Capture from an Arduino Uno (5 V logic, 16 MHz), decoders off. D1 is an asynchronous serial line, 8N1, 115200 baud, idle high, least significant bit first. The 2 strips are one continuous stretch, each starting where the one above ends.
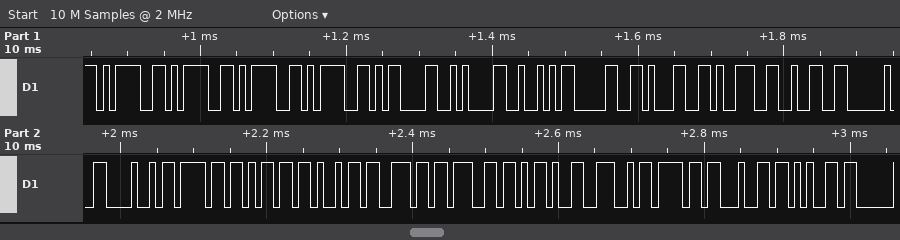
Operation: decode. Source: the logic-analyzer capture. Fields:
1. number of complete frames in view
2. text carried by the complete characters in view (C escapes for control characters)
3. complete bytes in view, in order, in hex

23
"====\r\nR0192 Homing-Node"
3D 3D 3D 3D 0D 0A 52 30 31 39 32 20 48 6F 6D 69 6E 67 2D 4E 6F 64 65
